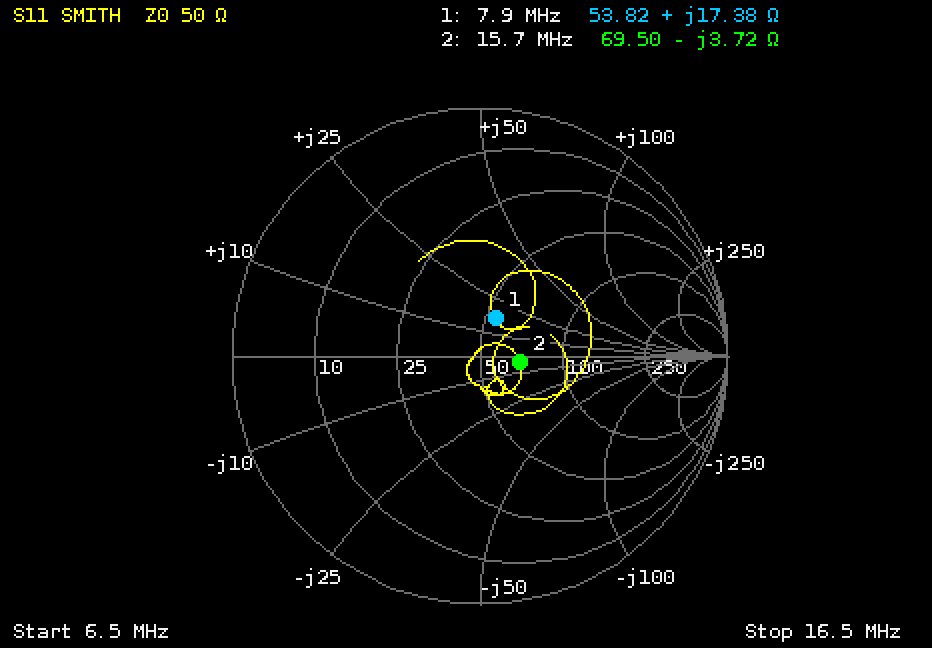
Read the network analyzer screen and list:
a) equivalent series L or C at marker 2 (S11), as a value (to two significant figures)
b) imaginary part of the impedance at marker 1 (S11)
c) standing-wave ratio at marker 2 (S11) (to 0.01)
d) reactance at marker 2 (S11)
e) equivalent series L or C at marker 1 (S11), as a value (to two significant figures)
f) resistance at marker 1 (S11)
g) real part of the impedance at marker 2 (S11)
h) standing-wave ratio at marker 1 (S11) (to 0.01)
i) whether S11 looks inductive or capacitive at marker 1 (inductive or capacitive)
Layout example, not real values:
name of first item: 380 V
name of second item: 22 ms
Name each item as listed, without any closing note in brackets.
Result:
equivalent series L or C at marker 2 (S11), as a value: 2.7 nF
imaginary part of the impedance at marker 1: +17.38 Ω
standing-wave ratio at marker 2 (S11): 1.40
reactance at marker 2: -3.72 Ω
equivalent series L or C at marker 1 (S11), as a value: 350 nH
resistance at marker 1: 53.82 Ω
real part of the impedance at marker 2: 69.50 Ω
standing-wave ratio at marker 1 (S11): 1.41
whether S11 looks inductive or capacitive at marker 1: inductive
